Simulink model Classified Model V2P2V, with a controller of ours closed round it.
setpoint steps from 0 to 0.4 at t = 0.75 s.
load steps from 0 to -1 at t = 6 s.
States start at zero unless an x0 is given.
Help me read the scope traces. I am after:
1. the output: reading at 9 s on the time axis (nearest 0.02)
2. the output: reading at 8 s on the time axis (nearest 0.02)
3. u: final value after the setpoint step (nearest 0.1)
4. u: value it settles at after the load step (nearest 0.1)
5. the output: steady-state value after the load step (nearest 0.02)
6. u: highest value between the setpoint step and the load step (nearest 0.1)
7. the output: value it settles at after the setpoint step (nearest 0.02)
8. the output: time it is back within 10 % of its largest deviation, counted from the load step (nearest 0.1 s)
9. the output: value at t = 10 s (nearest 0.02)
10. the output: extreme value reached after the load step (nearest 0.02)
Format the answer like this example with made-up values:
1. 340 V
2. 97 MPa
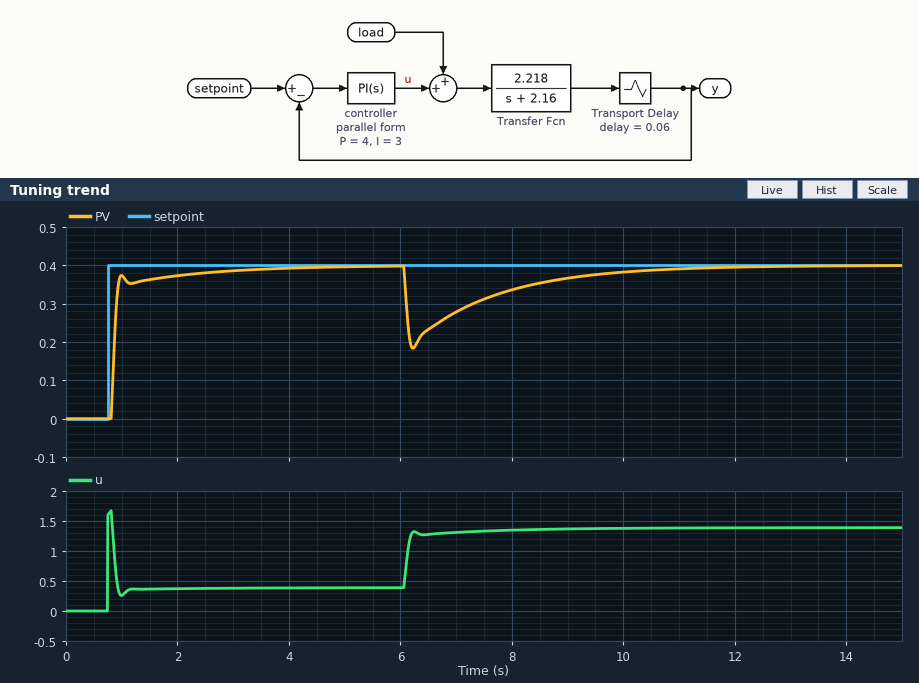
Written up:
1. 0.36
2. 0.34
3. 0.4
4. 1.4
5. 0.40
6. 1.7
7. 0.40
8. 3.7 s
9. 0.38
10. 0.18
